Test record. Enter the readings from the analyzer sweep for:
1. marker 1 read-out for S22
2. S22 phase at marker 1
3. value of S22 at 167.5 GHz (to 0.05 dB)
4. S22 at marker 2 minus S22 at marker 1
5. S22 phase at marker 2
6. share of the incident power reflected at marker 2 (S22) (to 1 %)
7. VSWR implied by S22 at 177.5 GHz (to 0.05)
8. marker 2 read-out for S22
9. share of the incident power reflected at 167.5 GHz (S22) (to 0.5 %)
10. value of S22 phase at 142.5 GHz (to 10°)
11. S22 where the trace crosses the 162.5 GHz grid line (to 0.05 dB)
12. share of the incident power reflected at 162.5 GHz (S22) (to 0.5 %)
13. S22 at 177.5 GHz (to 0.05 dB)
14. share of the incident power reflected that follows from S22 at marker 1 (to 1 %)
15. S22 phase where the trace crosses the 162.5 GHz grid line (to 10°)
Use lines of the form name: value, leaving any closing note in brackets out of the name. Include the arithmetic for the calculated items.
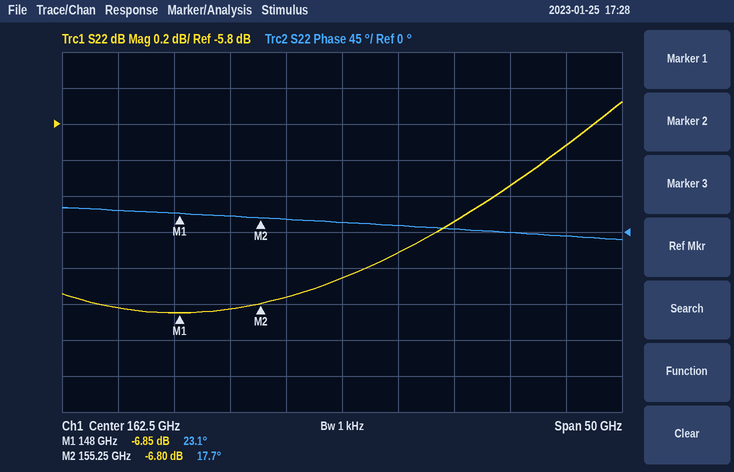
marker 1 read-out for S22: -6.85 dB
S22 phase at marker 1: 23.1°
value of S22 at 167.5 GHz: -6.50 dB
S22 at marker 2 minus S22 at marker 1: -6.8 − (-6.85) = 0.05 dB
S22 phase at marker 2: 17.7°
share of the incident power reflected at marker 2 (S22): 10^(-6.8/10) ≈ 21 %
VSWR implied by S22 at 177.5 GHz: |Γ| = 10^(-6.15/20) = 0.4926; VSWR = (1 + 0.4926)/(1 − 0.4926) ≈ 2.94, so 2.95 to the nearest 0.05
marker 2 read-out for S22: -6.80 dB
share of the incident power reflected at 167.5 GHz (S22): 10^(-6.5/10) ≈ 22.4 %, so 22.5 % to the nearest 0.5 %
value of S22 phase at 142.5 GHz: 30°
S22 where the trace crosses the 162.5 GHz grid line: -6.65 dB
share of the incident power reflected at 162.5 GHz (S22): 10^(-6.65/10) ≈ 21.6 %, so 21.5 % to the nearest 0.5 %
S22 at 177.5 GHz: -6.15 dB
share of the incident power reflected that follows from S22 at marker 1: 10^(-6.85/10) ≈ 21 %
S22 phase where the trace crosses the 162.5 GHz grid line: 10°
